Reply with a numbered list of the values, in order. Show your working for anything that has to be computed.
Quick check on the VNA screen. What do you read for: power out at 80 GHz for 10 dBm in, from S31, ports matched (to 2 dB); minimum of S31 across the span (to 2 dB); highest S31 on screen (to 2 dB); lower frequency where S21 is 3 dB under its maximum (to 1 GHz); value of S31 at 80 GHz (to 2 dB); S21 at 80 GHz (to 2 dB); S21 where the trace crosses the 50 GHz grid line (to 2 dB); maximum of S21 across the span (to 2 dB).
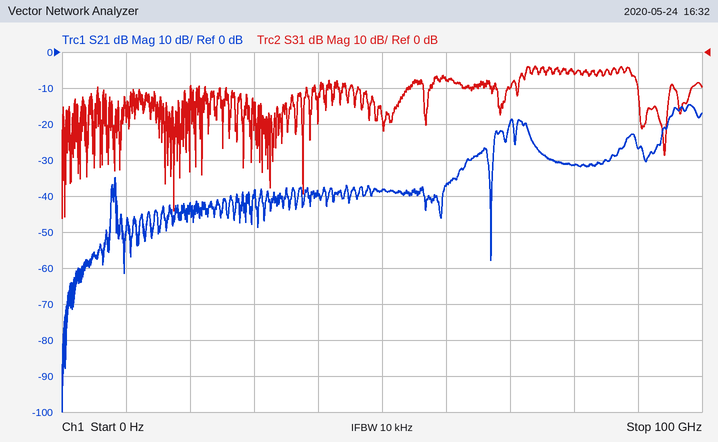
1. 10 dBm + (-6 dB) = 4 dBm
2. -46 dB
3. -4 dB
4. 95 GHz
5. -6 dB
6. -32 dB
7. -38 dB
8. -14 dB
